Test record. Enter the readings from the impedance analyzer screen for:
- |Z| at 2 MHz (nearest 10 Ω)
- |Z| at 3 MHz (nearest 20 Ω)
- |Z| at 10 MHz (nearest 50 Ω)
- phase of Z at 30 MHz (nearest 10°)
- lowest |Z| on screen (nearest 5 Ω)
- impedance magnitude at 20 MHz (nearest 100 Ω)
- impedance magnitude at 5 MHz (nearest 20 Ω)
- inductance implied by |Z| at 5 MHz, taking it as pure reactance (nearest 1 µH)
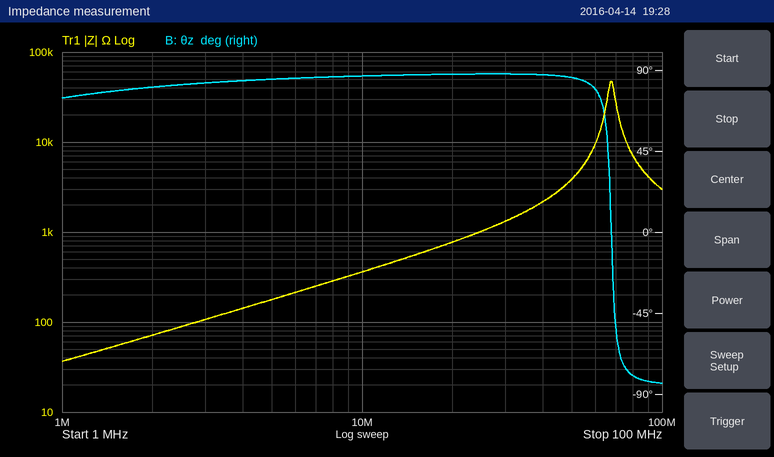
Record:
70 Ω
100 Ω
350 Ω
90°
35 Ω
800 Ω
180 Ω
6 µH
